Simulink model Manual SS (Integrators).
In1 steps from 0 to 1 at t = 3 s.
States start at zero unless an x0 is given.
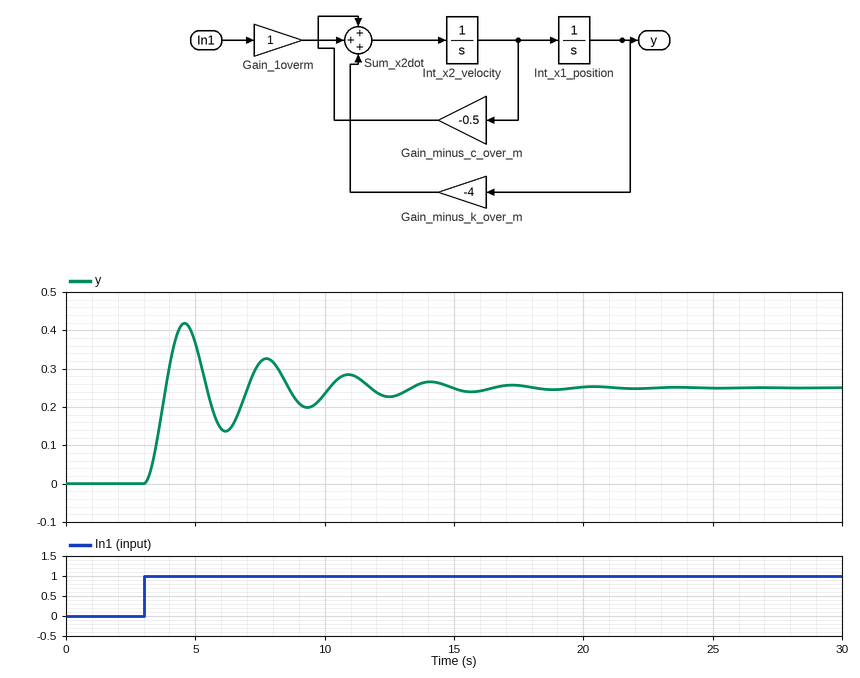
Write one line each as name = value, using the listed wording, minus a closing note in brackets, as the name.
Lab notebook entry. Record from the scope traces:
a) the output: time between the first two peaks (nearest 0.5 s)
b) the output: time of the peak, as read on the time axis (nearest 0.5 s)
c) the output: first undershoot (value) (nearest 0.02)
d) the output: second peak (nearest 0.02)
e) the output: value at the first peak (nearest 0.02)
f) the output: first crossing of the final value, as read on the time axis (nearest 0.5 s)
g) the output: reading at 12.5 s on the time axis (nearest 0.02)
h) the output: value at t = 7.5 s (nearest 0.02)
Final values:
the output: time between the first two peaks = 3.0 s
the output: time of the peak, as read on the time axis = 4.5 s
the output: first undershoot (value) = 0.14
the output: second peak = 0.32
the output: value at the first peak = 0.42
the output: first crossing of the final value, as read on the time axis = 4.0 s
the output: reading at 12.5 s on the time axis = 0.22
the output: value at t = 7.5 s = 0.32
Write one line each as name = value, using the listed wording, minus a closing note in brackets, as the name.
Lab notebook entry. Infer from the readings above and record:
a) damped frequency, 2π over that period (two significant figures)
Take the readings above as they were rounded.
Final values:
damped frequency, 2π over that period = 2.1 rad/s
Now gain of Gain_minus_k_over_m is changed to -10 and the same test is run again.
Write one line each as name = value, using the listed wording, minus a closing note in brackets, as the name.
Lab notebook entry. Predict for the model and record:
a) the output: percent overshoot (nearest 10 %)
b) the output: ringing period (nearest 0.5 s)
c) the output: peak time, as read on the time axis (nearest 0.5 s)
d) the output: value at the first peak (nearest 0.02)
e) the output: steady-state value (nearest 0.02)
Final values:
the output: percent overshoot = 80 %
the output: ringing period = 2.0 s
the output: peak time, as read on the time axis = 4.0 s
the output: value at the first peak = 0.18
the output: steady-state value = 0.10
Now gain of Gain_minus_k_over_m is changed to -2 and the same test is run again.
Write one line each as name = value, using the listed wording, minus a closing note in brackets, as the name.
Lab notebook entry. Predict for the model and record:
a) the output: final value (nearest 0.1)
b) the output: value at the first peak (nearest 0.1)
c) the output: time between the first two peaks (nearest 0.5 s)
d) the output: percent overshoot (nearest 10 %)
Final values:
the output: final value = 0.5
the output: value at the first peak = 0.8
the output: time between the first two peaks = 4.5 s
the output: percent overshoot = 60 %
